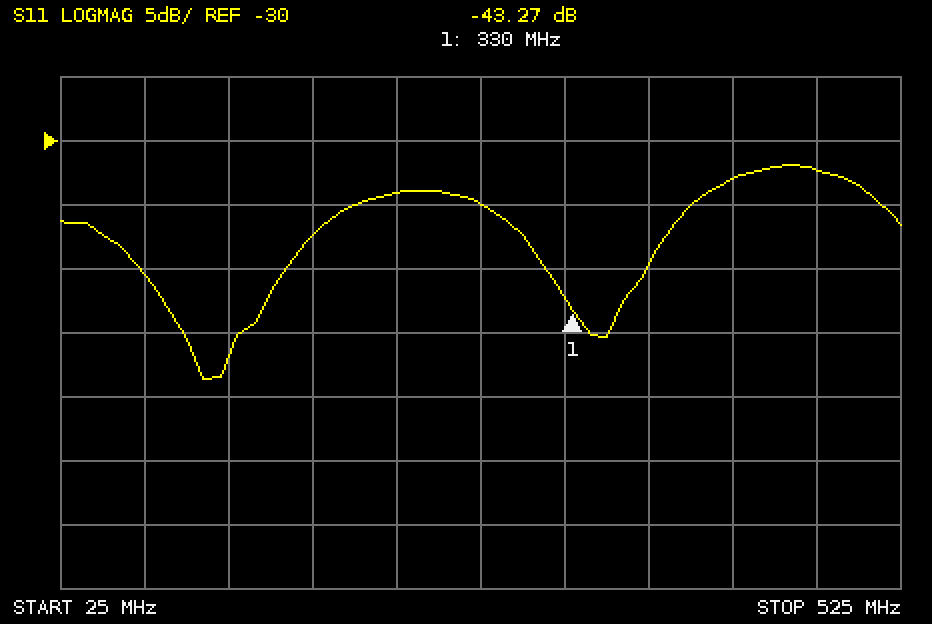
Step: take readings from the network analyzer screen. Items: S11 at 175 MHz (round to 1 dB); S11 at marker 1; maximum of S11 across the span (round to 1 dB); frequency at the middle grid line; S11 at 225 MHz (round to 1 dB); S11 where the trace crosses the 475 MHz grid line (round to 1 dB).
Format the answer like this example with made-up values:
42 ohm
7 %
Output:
-37 dB
-43.27 dB
-32 dB
275 MHz
-34 dB
-32 dB
